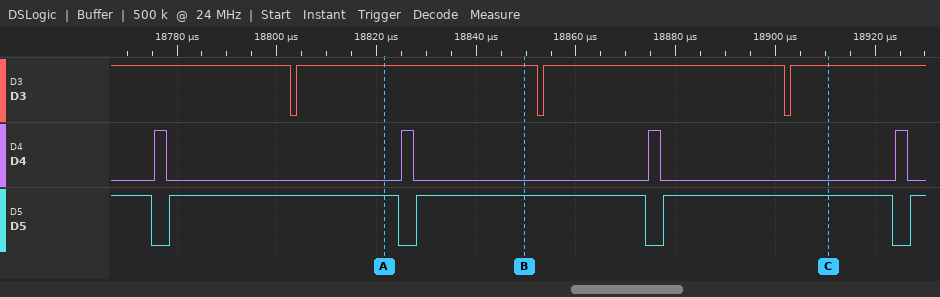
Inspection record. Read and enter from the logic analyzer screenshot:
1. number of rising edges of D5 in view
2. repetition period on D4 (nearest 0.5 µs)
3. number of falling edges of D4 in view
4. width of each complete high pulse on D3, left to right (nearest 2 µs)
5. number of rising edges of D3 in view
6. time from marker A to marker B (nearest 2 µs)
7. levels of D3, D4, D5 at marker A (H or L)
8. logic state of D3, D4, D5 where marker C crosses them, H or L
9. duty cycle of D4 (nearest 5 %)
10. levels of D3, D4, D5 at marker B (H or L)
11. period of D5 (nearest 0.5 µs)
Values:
4
49.5 µs
4
48 µs, 48 µs
3
28 µs
D3=H, D4=L, D5=H
D3=H, D4=L, D5=H
5 %
D3=H, D4=L, D5=H
49.5 µs
